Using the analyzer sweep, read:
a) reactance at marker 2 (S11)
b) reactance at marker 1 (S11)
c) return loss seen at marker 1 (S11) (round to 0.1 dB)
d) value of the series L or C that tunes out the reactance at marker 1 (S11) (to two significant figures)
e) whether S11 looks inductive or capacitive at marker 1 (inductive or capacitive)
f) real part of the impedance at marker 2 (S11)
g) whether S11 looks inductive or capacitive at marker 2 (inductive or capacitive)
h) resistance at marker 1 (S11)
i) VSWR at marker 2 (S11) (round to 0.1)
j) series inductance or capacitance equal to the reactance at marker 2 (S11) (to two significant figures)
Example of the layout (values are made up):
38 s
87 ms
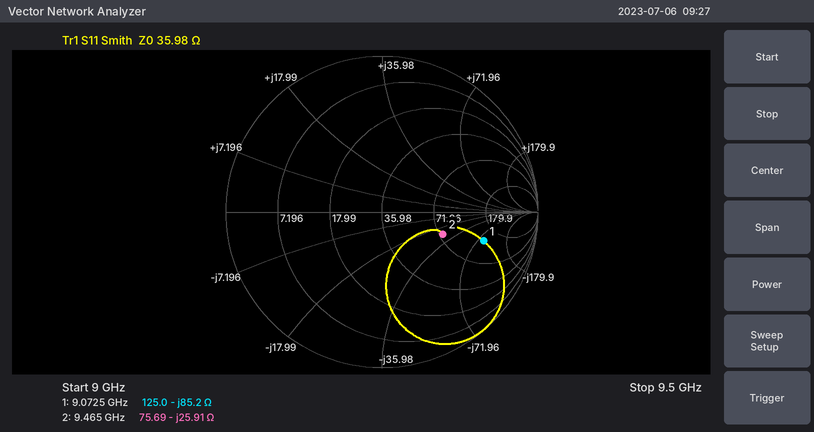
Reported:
-25.91 Ω
-85.2 Ω
3.4 dB
1.5 nH
capacitive
75.69 Ω
capacitive
125.0 Ω
2.4
650 fF
